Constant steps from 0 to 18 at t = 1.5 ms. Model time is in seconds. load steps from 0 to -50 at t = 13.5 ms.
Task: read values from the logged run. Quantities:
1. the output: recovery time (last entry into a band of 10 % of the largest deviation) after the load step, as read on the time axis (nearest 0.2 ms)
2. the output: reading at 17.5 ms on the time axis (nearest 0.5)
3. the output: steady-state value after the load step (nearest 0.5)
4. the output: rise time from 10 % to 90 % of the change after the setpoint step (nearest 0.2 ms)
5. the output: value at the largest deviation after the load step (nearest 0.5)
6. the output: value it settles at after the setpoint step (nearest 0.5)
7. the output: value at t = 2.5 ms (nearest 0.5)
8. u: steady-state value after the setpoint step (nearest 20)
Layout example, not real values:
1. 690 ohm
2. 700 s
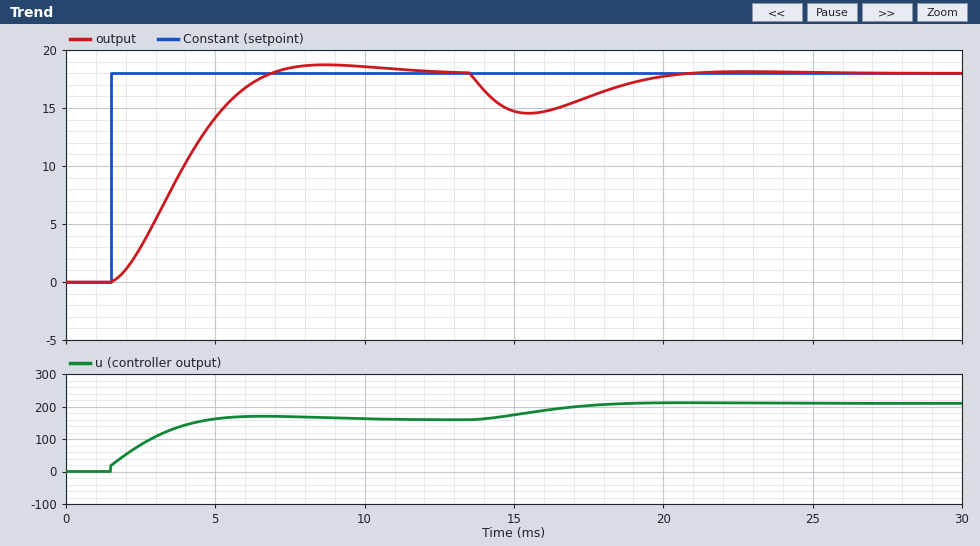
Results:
1. 19.8 ms
2. 16.0
3. 18.0
4. 3.6 ms
5. 14.5
6. 18.0
7. 3.0
8. 160
